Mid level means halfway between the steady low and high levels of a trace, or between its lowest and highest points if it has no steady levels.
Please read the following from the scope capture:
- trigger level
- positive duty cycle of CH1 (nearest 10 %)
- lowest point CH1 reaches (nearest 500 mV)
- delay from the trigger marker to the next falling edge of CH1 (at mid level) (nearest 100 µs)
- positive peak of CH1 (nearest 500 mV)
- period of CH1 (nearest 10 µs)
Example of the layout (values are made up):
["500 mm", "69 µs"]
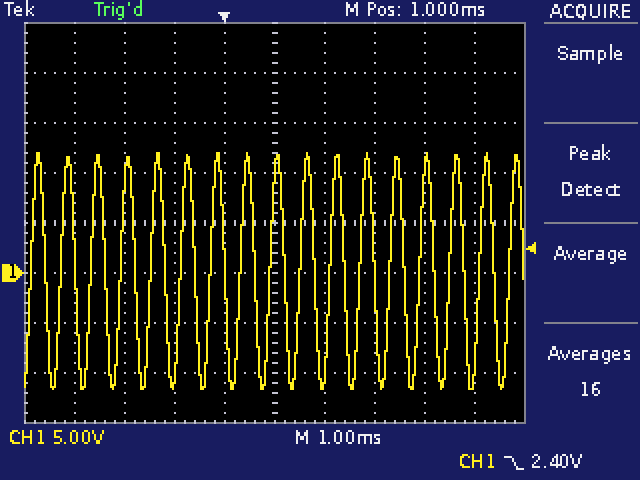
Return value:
["2.40 V", "50 %", "-11.5 V", "600 µs", "12.0 V", "600 µs"]
